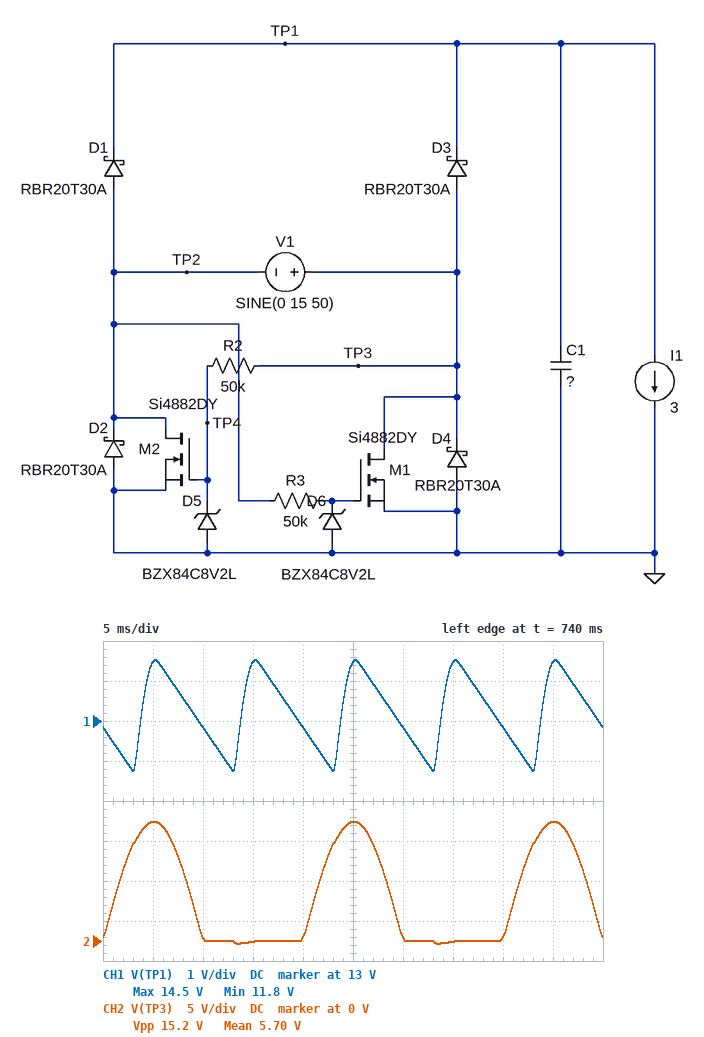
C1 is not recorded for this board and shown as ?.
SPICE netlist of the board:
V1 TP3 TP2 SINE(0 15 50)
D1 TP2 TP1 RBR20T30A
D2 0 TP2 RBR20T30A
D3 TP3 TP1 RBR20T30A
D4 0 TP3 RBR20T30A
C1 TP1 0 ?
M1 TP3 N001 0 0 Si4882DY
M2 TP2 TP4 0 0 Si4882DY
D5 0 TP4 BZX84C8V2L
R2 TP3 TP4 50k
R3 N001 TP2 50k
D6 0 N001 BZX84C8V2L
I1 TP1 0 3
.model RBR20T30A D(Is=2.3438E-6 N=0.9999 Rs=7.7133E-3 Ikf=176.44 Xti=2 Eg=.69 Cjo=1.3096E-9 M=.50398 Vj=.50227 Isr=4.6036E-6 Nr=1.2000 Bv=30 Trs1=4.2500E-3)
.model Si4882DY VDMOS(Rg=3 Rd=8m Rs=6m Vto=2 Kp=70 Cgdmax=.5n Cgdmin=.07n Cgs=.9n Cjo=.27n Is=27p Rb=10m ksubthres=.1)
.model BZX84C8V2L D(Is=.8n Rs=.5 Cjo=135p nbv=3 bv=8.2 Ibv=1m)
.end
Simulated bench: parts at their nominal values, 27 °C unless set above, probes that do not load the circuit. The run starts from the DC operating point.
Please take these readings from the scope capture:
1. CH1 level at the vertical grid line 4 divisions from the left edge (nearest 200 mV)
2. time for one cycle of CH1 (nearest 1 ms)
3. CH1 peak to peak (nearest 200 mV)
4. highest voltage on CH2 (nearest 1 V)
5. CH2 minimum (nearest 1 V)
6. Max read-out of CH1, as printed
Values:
12.8 V
10 ms
2.8 V
15 V
0 V
14.5 V
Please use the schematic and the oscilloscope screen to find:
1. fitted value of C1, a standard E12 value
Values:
8.2 mF
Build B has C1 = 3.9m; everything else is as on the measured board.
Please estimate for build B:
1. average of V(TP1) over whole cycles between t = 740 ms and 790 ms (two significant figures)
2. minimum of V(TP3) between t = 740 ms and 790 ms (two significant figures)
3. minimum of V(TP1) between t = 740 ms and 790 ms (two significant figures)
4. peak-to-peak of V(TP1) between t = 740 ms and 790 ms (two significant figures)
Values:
12 V
-250 mV
9.3 V
5.2 V
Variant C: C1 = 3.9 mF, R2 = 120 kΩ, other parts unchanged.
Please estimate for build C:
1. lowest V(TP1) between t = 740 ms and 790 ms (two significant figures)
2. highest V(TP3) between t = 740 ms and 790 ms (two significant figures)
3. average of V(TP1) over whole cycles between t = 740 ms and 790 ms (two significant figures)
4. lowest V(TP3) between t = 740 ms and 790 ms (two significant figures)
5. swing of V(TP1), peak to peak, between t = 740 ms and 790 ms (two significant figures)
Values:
9.3 V
15 V
12 V
-250 mV
5.2 V
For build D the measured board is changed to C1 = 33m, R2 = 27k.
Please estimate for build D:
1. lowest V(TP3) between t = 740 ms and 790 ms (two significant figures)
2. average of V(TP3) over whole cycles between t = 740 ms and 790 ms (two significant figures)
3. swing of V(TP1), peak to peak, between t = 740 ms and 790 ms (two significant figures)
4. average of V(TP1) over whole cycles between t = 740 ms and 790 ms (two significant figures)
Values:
-370 mV
4.7 V
740 mV
14 V
